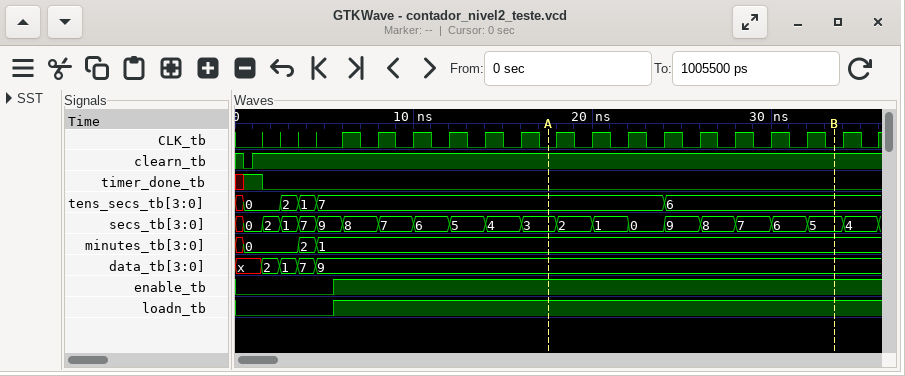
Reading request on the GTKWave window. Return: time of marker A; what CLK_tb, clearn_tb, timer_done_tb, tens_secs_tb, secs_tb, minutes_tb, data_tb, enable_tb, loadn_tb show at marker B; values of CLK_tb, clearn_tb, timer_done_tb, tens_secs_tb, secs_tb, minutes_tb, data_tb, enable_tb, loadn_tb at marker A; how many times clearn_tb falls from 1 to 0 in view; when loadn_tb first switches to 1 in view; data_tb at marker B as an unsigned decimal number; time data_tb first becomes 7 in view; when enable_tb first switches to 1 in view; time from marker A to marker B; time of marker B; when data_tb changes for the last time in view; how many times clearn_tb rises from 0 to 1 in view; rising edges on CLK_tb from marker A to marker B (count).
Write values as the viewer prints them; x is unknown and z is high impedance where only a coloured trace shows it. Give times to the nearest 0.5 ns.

17.5 ns
CLK_tb=0, clearn_tb=1, timer_done_tb=0, tens_secs_tb=6, secs_tb=5, minutes_tb=1, data_tb=9, enable_tb=1, loadn_tb=1
CLK_tb=0, clearn_tb=1, timer_done_tb=0, tens_secs_tb=7, secs_tb=3, minutes_tb=1, data_tb=9, enable_tb=1, loadn_tb=1
1
5.5 ns
9
3.5 ns
5.5 ns
16 ns
33.5 ns
4.5 ns
1
8
